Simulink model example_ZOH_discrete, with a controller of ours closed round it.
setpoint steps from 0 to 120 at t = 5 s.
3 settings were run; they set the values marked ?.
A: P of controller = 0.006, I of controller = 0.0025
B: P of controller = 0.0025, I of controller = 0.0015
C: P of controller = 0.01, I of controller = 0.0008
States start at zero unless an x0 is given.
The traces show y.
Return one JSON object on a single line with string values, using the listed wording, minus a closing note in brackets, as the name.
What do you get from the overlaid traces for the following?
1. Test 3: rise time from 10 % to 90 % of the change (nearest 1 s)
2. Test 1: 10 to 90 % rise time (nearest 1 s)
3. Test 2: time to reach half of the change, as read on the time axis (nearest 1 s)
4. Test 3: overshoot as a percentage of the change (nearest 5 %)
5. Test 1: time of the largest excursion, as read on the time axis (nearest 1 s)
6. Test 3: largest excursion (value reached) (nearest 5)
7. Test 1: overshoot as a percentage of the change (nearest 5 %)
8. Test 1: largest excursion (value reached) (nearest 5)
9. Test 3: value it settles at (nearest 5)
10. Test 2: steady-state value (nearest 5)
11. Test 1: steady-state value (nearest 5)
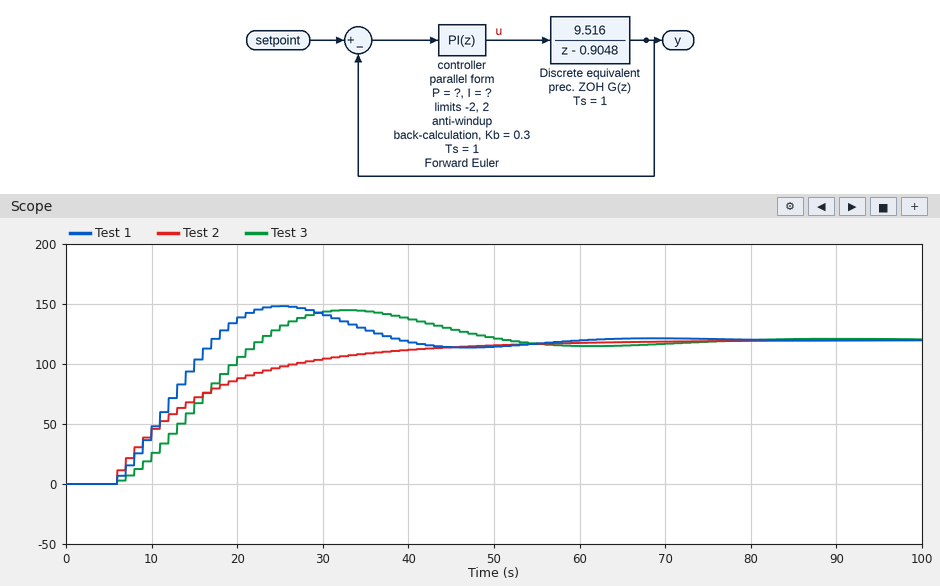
{"Test 3: rise time from 10 % to 90 % of the change": "13 s", "Test 1: 10 to 90 % rise time": "9 s", "Test 2: time to reach half of the change, as read on the time axis": "13 s", "Test 3: overshoot as a percentage of the change": "20 %", "Test 1: time of the largest excursion, as read on the time axis": "25 s", "Test 3: largest excursion (value reached)": "145", "Test 1: overshoot as a percentage of the change": "25 %", "Test 1: largest excursion (value reached)": "150", "Test 3: value it settles at": "120", "Test 2: steady-state value": "120", "Test 1: steady-state value": "120"}
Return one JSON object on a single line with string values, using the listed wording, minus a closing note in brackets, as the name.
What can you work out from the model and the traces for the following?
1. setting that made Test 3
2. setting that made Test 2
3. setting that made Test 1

{"setting that made Test 3": "B", "setting that made Test 2": "C", "setting that made Test 1": "A"}
